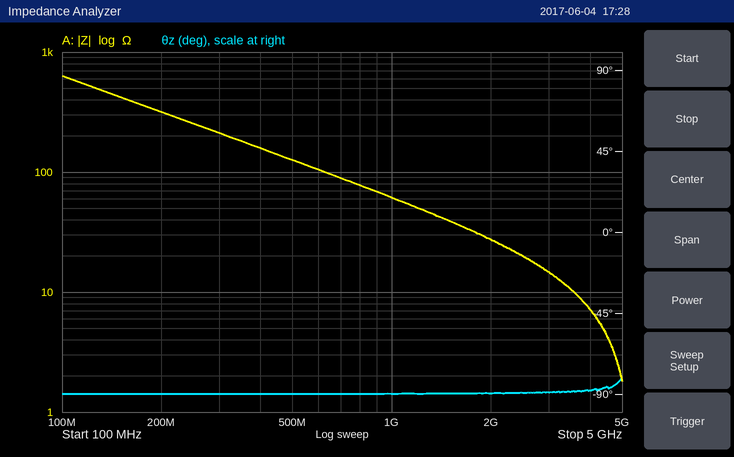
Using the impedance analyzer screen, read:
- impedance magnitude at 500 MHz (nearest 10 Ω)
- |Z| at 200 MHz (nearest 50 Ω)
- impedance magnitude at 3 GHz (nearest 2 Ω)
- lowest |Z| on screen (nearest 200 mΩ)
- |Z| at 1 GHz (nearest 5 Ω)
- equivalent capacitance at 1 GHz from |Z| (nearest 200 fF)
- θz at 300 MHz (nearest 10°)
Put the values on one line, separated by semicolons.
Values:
130 Ω; 300 Ω; 14 Ω; 1.8 Ω; 60 Ω; 2.6 pF; -90°
